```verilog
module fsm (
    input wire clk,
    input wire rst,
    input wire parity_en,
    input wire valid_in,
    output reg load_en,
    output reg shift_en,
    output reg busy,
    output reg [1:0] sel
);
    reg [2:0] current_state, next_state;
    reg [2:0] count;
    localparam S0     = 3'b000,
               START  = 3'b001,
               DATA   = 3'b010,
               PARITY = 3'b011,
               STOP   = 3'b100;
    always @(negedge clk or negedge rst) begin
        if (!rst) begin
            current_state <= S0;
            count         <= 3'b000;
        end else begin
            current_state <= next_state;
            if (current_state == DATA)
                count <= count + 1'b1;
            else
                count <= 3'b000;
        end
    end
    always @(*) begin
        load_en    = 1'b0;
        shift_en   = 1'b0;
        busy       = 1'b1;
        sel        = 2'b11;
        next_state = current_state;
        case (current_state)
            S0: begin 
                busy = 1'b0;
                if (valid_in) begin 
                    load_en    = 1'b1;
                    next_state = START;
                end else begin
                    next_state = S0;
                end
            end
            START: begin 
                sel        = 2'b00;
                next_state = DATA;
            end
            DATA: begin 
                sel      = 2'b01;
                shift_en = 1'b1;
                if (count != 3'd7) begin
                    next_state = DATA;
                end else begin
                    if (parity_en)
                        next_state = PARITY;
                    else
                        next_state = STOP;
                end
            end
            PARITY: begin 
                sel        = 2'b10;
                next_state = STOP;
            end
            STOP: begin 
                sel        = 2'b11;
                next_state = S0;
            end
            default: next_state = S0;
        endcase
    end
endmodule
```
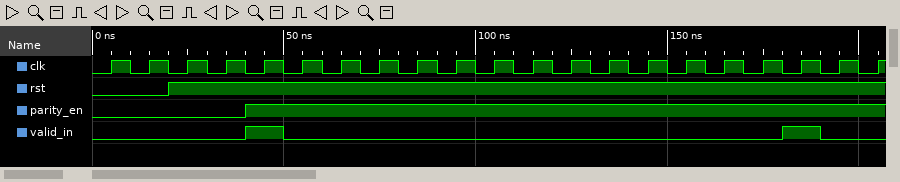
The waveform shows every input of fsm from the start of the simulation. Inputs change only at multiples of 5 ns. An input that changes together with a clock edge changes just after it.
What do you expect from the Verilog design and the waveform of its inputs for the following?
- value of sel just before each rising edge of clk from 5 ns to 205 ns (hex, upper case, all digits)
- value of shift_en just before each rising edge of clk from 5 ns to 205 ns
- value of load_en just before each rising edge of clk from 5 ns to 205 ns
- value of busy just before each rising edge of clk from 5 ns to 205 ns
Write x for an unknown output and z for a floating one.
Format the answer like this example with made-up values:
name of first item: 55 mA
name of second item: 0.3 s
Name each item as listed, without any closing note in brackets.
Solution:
value of sel just before each rising edge of clk from 5 ns to 205 ns: 3, 3, 3, 3, 3, 0, 1, 1, 1, 1, 1, 1, 1, 1, 2, 3, 3, 3, 3, 0, 1
value of shift_en just before each rising edge of clk from 5 ns to 205 ns: 0 0 0 0 0 0 1 1 1 1 1 1 1 1 0 0 0 0 0 0 1
value of load_en just before each rising edge of clk from 5 ns to 205 ns: 0 0 0 0 1 0 0 0 0 0 0 0 0 0 0 0 0 0 1 0 0
value of busy just before each rising edge of clk from 5 ns to 205 ns: 0 0 0 0 0 1 1 1 1 1 1 1 1 1 1 1 0 0 0 1 1
